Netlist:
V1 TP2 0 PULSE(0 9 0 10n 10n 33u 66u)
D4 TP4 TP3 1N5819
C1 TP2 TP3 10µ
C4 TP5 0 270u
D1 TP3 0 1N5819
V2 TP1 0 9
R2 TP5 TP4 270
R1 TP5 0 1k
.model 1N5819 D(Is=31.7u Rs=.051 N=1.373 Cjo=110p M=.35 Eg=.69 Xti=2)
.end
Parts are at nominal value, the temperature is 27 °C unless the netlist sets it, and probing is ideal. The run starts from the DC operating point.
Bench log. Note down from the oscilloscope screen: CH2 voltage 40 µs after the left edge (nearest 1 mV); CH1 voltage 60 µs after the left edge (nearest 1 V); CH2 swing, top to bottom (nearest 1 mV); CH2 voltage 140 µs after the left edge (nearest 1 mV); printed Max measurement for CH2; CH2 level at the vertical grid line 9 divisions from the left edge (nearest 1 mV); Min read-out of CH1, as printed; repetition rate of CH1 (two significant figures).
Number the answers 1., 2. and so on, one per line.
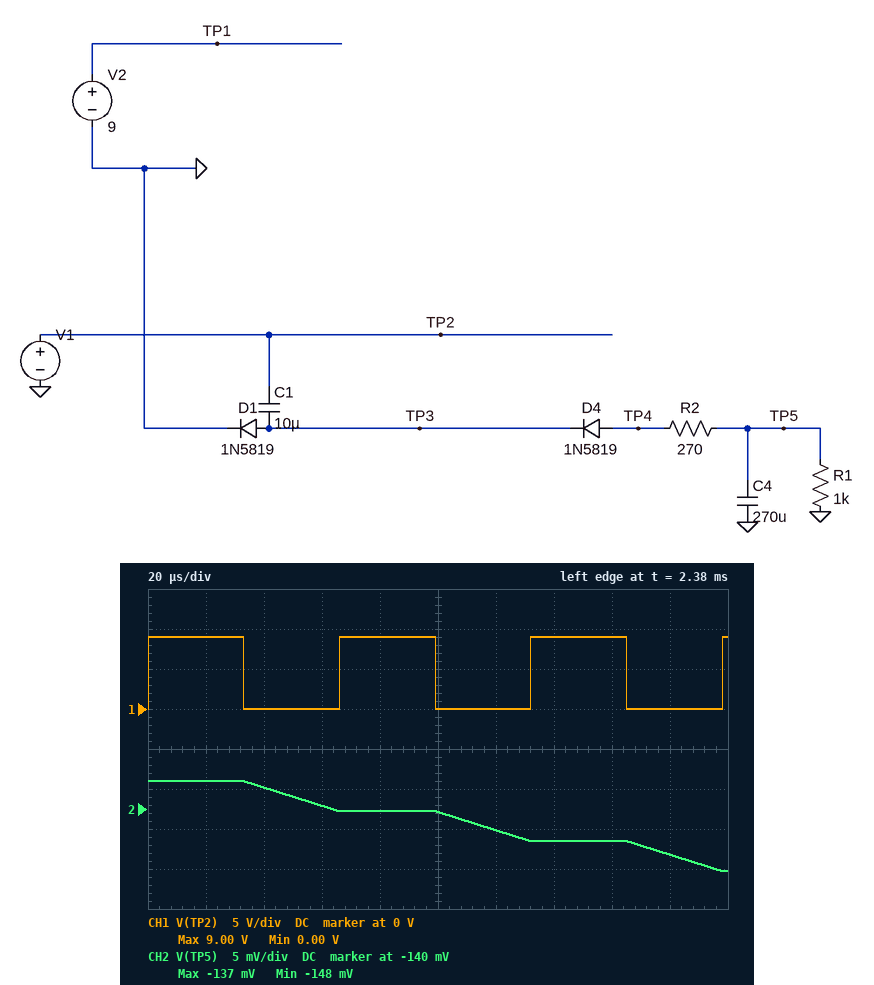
1. -137 mV
2. 0 V
3. 11 mV
4. -144 mV
5. -137 mV
6. -146 mV
7. 0.00 V
8. 15 kHz
